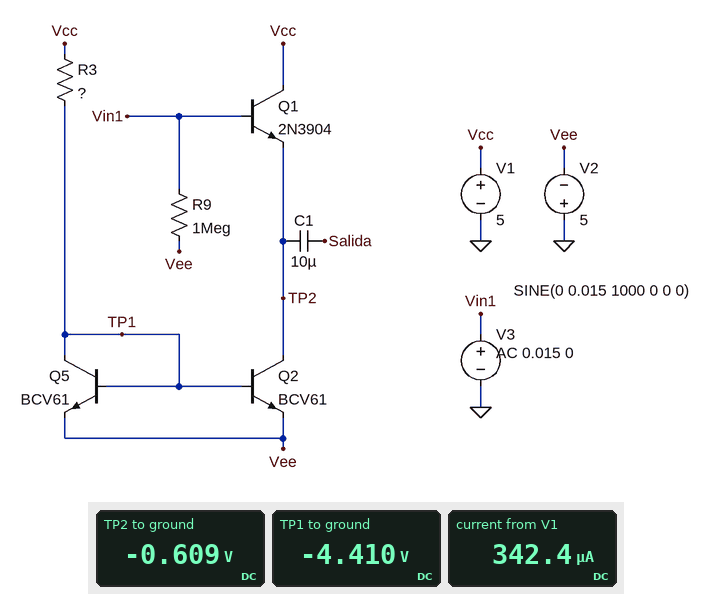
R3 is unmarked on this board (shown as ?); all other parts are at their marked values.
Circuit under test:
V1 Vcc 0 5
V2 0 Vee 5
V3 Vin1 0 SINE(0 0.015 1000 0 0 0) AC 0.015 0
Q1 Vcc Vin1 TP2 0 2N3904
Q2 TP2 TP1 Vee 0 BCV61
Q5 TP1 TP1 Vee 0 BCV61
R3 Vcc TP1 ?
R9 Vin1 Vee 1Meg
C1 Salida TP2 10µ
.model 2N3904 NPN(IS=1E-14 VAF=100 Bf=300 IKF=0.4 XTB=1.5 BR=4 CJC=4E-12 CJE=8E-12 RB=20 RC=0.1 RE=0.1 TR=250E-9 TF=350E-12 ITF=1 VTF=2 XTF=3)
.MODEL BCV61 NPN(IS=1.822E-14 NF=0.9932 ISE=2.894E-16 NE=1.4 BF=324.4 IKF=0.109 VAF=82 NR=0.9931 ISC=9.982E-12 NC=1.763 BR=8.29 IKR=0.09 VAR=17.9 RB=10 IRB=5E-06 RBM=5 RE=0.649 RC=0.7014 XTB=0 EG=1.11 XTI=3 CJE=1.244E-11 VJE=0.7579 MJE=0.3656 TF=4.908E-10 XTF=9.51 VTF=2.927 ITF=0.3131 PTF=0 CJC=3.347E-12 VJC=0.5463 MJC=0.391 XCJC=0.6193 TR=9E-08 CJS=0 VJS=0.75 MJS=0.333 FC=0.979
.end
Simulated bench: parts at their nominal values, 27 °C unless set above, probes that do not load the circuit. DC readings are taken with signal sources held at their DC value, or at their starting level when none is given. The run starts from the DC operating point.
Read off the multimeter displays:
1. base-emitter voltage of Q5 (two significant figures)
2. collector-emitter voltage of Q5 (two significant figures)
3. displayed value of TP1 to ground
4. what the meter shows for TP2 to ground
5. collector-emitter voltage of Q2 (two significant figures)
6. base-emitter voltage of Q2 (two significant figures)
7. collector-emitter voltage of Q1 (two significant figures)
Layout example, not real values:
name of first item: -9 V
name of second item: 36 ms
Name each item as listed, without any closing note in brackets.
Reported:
base-emitter voltage of Q5: 590 mV
collector-emitter voltage of Q5: 590 mV
displayed value of TP1 to ground: -4.410 V
what the meter shows for TP2 to ground: -0.609 V
collector-emitter voltage of Q2: 4.4 V
base-emitter voltage of Q2: 590 mV
collector-emitter voltage of Q1: 5.6 V
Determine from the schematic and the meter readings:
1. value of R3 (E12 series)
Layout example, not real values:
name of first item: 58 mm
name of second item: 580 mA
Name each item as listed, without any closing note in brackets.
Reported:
value of R3: 56 kΩ
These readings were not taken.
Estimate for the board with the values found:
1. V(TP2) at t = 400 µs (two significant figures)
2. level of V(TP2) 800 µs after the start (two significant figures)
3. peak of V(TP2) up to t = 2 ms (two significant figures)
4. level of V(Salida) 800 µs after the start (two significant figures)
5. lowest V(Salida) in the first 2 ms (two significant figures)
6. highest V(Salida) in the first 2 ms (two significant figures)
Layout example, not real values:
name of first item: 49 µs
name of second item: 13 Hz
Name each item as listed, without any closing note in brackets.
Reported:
V(TP2) at t = 400 µs: -600 mV
level of V(TP2) 800 µs after the start: -620 mV
peak of V(TP2) up to t = 2 ms: -590 mV
level of V(Salida) 800 µs after the start: -14 mV
lowest V(Salida) in the first 2 ms: -15 mV
highest V(Salida) in the first 2 ms: 15 mV
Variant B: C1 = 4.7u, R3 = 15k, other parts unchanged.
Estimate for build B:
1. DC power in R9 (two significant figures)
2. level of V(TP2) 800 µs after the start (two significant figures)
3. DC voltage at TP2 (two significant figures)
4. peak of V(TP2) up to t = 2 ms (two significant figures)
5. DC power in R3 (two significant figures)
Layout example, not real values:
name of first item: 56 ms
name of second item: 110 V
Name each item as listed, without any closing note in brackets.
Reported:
DC power in R9: 25 µW
level of V(TP2) 800 µs after the start: -660 mV
DC voltage at TP2: -640 mV
peak of V(TP2) up to t = 2 ms: -630 mV
DC power in R3: 5.9 mW
